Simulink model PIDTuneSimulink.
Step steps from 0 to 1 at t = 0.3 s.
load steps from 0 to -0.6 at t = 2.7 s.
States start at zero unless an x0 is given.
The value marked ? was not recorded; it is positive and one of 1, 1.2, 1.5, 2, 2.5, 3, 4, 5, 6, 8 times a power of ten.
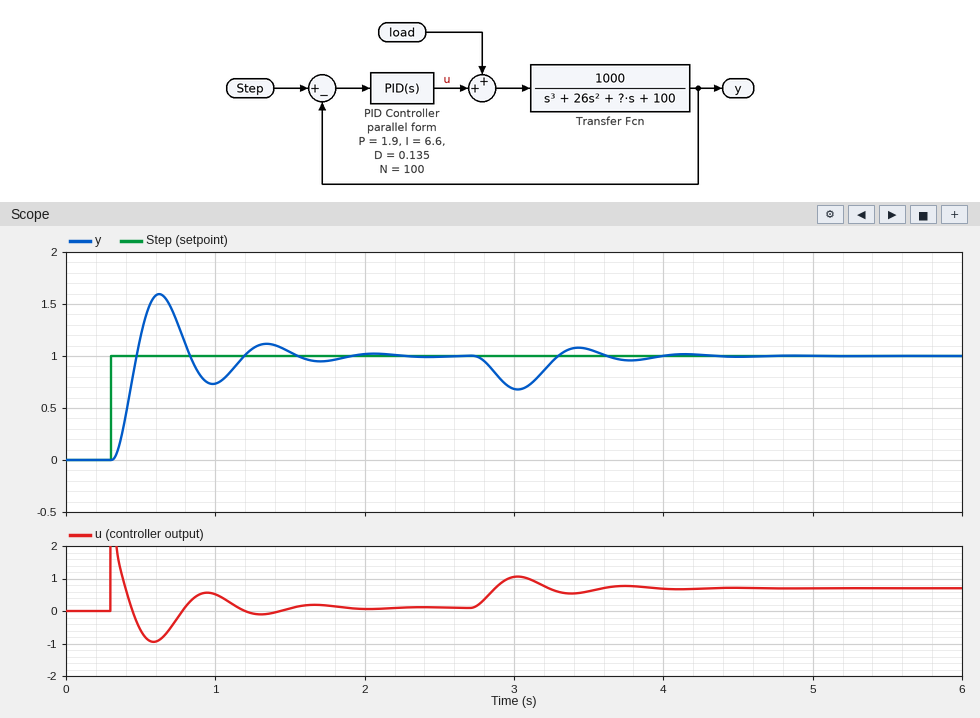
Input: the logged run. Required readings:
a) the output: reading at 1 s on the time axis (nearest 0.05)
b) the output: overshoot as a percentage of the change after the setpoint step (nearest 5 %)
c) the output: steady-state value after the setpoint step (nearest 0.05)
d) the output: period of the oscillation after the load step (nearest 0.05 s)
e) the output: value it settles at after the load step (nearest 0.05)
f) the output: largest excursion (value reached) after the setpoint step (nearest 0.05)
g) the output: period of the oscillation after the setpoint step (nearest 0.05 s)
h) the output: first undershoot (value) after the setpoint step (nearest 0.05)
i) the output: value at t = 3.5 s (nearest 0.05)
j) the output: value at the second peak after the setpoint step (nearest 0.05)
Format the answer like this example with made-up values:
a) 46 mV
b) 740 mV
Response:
a) 0.75
b) 60 %
c) 1.00
d) 0.75 s
e) 1.00
f) 1.60
g) 0.70 s
h) 0.75
i) 1.05
j) 1.10
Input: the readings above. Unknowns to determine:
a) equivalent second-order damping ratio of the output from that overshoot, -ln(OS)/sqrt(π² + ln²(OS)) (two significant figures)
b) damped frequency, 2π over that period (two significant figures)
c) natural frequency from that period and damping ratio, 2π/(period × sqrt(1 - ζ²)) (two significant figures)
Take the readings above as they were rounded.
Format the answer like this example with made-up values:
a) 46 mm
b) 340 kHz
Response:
a) 0.16
b) 9.0 rad/s
c) 9.1 rad/s
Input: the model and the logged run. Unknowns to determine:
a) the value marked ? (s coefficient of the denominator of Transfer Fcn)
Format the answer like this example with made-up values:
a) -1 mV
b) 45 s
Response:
a) 120
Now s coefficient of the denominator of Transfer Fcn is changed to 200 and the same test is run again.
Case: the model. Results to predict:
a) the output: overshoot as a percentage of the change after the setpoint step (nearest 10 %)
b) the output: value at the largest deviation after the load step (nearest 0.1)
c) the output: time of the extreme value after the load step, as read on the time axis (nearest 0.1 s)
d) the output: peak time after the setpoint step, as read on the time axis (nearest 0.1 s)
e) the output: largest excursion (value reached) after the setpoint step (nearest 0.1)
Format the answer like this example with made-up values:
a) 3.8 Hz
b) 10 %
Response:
a) 40 %
b) 0.7
c) 3.0 s
d) 0.6 s
e) 1.4
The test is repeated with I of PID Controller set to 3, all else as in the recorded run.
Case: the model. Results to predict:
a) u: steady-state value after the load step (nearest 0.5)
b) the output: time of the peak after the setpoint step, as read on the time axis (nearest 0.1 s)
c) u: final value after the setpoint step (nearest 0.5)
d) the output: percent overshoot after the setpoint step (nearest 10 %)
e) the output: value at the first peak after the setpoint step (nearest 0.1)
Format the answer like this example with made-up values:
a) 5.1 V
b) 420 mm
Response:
a) 0.5
b) 0.6 s
c) 0.0
d) 40 %
e) 1.4
